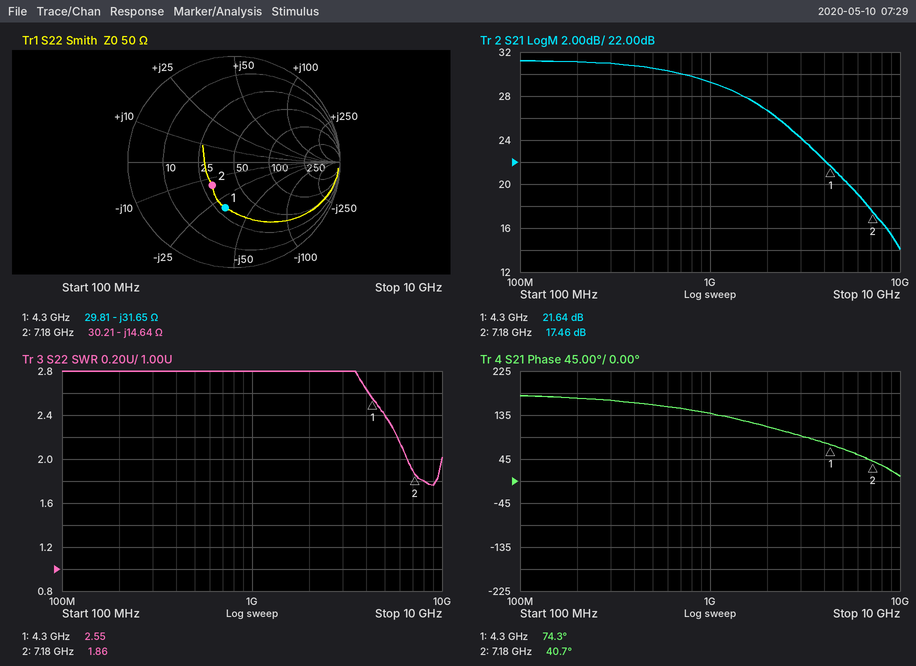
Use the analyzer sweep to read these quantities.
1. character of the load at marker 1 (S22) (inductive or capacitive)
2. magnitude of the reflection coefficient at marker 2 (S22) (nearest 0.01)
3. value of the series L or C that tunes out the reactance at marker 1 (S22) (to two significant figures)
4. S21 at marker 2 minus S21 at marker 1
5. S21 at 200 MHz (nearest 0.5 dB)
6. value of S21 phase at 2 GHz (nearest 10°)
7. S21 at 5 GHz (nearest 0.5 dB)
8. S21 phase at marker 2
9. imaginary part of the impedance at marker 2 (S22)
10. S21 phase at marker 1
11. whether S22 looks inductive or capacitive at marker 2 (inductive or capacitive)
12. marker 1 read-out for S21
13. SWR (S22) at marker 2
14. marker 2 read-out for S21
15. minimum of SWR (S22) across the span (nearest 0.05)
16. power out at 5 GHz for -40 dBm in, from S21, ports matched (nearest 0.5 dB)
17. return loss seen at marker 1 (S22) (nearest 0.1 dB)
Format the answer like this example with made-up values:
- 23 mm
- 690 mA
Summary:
- capacitive
- 0.30
- 1.2 nH
- -4.18 dB
- 31.0 dB
- 110°
- 20.5 dB
- 40.7°
- -14.64 Ω
- 74.3°
- capacitive
- 21.64 dB
- 1.86
- 17.46 dB
- 1.75
- -19.5 dBm
- 7.2 dB
